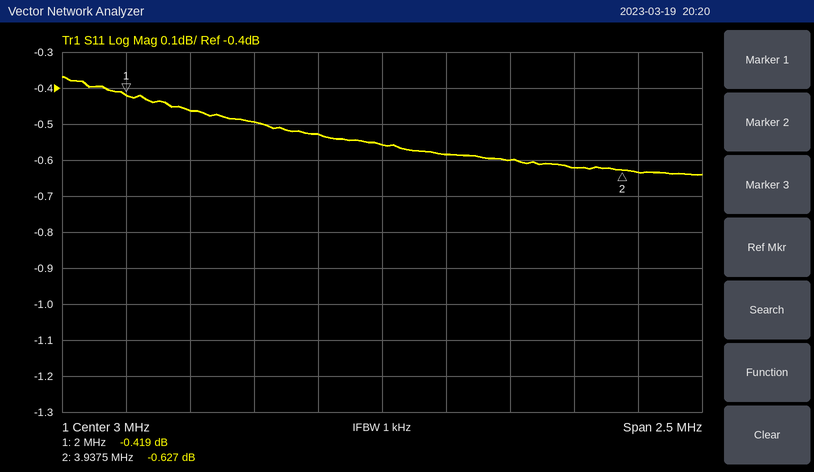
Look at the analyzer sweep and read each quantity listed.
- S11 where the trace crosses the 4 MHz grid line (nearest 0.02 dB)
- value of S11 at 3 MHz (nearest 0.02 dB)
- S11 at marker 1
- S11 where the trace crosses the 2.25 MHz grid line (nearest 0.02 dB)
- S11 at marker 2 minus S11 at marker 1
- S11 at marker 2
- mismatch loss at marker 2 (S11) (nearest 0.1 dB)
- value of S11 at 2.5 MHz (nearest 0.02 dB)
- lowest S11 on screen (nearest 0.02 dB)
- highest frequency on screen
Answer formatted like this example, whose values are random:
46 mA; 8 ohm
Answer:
-0.64 dB; -0.56 dB; -0.419 dB; -0.46 dB; -0.208 dB; -0.627 dB; 8.7 dB; -0.50 dB; -0.64 dB; 4.25 MHz
